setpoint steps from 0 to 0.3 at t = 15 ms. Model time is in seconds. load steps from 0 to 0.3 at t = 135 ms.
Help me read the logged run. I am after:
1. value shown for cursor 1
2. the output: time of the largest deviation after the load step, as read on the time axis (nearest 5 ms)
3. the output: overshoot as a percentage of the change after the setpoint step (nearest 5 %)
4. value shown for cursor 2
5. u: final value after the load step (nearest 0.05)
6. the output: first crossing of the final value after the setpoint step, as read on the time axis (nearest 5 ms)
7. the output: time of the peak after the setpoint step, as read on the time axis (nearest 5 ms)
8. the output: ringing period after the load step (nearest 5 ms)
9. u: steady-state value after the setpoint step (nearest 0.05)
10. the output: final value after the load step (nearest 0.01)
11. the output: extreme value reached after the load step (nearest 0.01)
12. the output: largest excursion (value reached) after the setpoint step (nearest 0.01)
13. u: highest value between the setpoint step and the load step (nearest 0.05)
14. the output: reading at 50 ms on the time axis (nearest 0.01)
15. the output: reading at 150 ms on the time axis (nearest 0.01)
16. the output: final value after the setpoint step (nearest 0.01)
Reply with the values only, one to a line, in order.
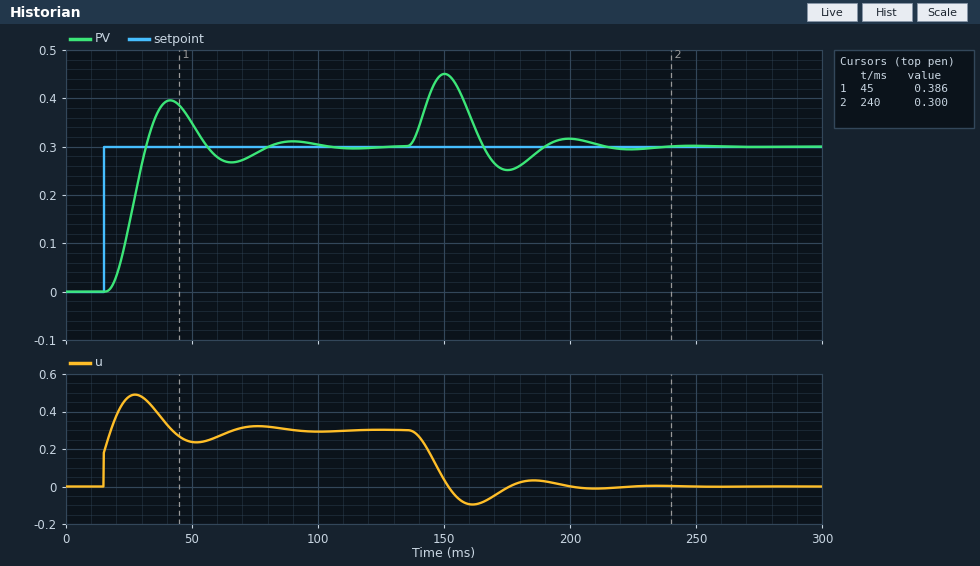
0.386
150 ms
30 %
0.300
0.00
30 ms
40 ms
50 ms
0.30
0.30
0.45
0.40
0.50
0.35
0.45
0.30
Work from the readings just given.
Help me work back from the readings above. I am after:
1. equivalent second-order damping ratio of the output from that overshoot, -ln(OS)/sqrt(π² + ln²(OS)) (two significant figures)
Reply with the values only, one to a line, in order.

0.36
